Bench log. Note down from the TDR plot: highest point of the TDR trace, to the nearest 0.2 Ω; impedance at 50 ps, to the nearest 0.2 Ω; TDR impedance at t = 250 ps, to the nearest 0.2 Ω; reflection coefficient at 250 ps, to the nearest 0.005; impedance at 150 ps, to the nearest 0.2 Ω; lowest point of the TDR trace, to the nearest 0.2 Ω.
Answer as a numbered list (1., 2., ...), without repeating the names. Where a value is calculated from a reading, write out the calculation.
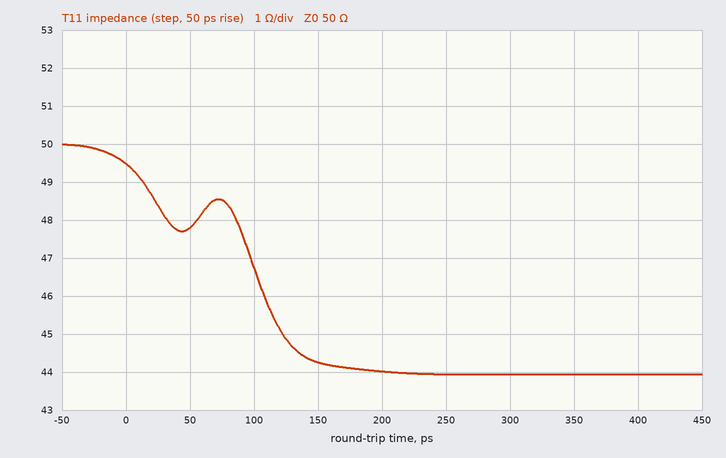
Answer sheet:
1. 50.0 Ω
2. 47.8 Ω
3. 44.0 Ω
4. (44 − 50)/(44 + 50) ≈ -0.0638, so -0.065 to the nearest 0.005
5. 44.2 Ω
6. 44.0 Ω
